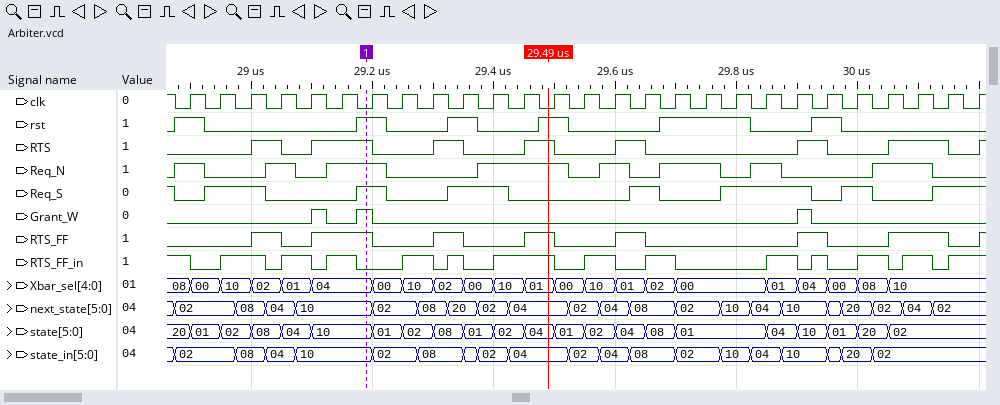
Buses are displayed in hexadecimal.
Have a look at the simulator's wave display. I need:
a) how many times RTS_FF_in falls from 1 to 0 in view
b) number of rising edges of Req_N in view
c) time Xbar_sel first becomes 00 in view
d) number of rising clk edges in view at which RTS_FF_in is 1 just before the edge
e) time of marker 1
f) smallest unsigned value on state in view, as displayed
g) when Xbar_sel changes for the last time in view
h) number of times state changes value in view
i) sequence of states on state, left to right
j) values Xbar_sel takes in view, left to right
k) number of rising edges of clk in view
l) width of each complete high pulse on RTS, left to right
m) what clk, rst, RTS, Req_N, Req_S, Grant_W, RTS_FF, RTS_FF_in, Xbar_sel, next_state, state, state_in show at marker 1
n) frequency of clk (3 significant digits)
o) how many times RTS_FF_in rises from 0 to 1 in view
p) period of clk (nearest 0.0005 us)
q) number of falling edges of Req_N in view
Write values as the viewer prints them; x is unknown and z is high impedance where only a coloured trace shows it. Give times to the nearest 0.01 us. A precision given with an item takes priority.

13
8
28.9 us
15
29.19 us
01
30.05 us
21
20, 01, 02, 08, 04, 10, 01, 02, 08, 01, 02, 04, 01, 02, 04, 08, 01, 04, 10, 01, 20, 02
08, 00, 10, 02, 01, 04, 00, 10, 02, 00, 10, 01, 00, 10, 01, 02, 00, 01, 04, 00, 08, 10
27
0.05 us, 0.1 us, 0.05 us, 0.05 us, 0.05 us, 0.05 us, 0.1 us
clk=0, rst=1, RTS=1, Req_N=1, Req_S=1, Grant_W=1, RTS_FF=1, RTS_FF_in=0, Xbar_sel=04, next_state=10, state=10, state_in=10
20.0 MHz
13
0.05 us
8
